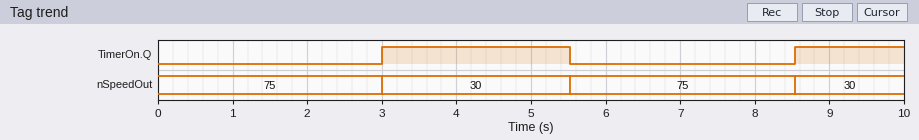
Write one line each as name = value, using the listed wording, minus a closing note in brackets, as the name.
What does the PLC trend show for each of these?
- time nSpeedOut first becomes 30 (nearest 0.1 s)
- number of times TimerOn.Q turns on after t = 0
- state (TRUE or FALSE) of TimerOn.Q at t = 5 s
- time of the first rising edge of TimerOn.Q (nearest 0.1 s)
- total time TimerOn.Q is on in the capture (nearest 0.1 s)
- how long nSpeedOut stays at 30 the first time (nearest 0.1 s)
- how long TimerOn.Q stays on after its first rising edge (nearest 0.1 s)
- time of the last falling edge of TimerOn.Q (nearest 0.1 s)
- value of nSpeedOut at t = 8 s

time nSpeedOut first becomes 30 = 3.0 s
number of times TimerOn.Q turns on after t = 0 = 2
state (TRUE or FALSE) of TimerOn.Q at t = 5 s = TRUE
time of the first rising edge of TimerOn.Q = 3.0 s
total time TimerOn.Q is on in the capture = 4.0 s
how long nSpeedOut stays at 30 the first time = 2.5 s
how long TimerOn.Q stays on after its first rising edge = 2.5 s
time of the last falling edge of TimerOn.Q = 5.5 s
value of nSpeedOut at t = 8 s = 75
